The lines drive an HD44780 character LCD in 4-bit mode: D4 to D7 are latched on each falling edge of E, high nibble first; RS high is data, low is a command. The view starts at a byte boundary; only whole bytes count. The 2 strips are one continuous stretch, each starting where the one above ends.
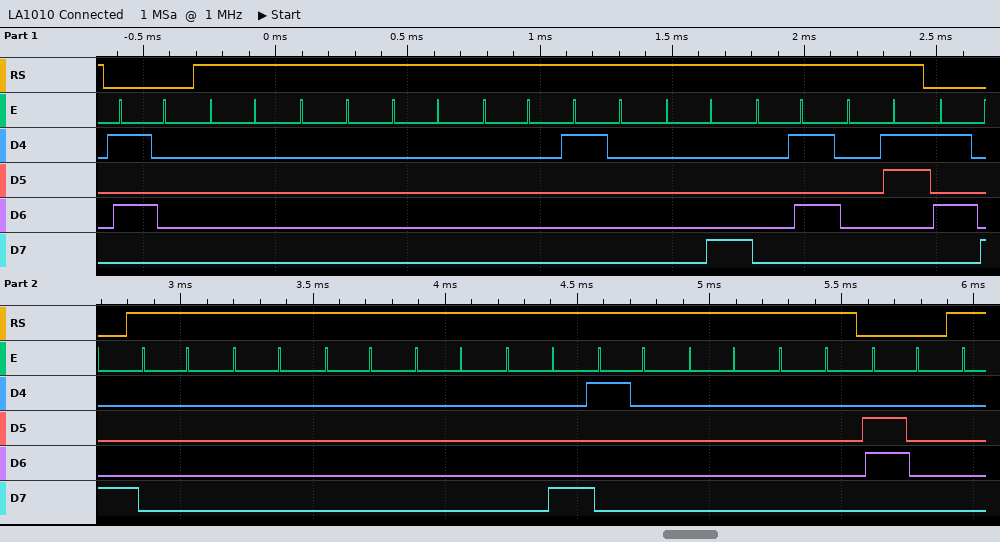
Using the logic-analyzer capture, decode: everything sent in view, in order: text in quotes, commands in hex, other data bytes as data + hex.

0x50 data 00 00 00 00 10 08 05 03 0x58 data 00 00 00 00 08 10 00 00 0x60
